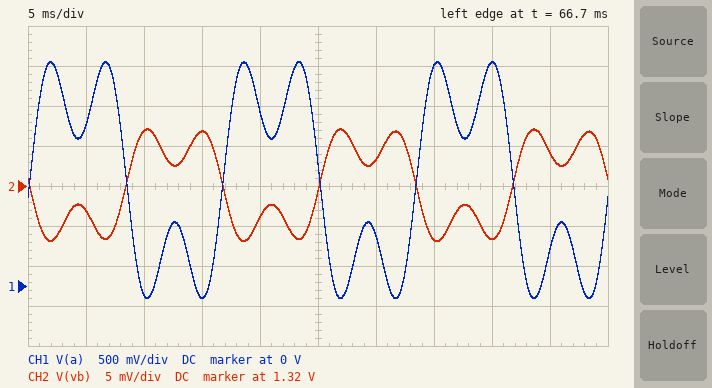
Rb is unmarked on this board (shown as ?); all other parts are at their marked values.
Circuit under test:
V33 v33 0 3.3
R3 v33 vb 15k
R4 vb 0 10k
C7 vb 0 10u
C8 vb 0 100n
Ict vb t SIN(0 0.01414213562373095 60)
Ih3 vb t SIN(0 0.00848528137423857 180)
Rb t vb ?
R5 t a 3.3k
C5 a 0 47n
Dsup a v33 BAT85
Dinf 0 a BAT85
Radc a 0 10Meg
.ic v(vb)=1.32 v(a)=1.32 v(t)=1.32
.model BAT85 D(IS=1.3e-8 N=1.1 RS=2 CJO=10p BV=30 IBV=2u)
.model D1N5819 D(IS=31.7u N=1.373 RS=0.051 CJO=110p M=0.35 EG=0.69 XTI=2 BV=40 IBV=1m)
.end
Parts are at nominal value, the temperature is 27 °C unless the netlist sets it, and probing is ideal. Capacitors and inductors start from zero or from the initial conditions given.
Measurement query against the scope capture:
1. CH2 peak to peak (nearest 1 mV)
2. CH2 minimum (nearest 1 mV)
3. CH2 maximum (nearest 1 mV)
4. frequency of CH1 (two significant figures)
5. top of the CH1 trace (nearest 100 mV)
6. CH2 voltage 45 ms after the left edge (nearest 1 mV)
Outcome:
14 mV
1.313 V
1.327 V
60 Hz
2.8 V
1.324 V
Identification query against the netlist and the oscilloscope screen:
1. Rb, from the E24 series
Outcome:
91 Ω
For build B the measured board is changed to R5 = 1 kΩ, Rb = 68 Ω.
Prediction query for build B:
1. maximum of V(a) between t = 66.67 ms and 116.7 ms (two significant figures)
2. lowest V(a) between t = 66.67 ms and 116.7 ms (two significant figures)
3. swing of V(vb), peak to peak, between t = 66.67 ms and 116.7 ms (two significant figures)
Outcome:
2.4 V
210 mV
11 mV
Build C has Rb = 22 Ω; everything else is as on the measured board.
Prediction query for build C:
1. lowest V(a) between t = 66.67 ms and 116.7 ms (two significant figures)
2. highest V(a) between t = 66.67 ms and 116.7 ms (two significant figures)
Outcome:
960 mV
1.7 V
